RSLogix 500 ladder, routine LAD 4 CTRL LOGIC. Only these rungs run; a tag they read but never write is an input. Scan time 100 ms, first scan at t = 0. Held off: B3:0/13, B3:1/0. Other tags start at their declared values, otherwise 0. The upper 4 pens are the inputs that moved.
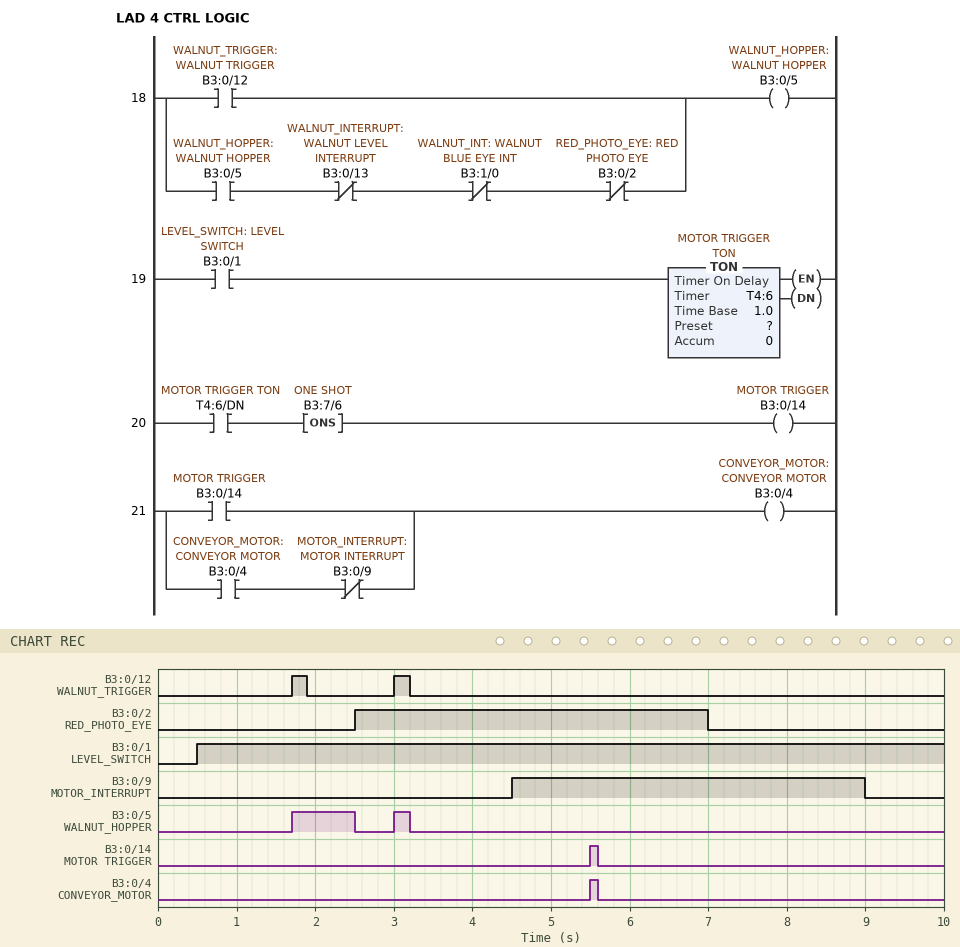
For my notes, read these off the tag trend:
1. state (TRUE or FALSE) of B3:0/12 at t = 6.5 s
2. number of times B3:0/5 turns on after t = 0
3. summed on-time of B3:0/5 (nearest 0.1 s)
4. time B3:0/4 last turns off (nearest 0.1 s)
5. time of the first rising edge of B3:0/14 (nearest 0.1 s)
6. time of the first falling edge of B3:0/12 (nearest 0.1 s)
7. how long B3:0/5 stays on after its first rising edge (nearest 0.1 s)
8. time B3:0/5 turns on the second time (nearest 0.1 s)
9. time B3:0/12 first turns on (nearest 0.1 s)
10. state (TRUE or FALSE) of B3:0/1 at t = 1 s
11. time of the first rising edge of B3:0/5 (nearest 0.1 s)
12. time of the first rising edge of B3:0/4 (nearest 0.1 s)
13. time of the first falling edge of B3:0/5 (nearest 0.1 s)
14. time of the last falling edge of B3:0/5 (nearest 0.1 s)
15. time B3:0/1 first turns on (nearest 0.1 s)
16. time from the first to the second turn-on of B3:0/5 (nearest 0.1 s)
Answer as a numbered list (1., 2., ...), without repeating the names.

1. FALSE
2. 2
3. 1.0 s
4. 5.6 s
5. 5.5 s
6. 1.9 s
7. 0.8 s
8. 3.0 s
9. 1.7 s
10. TRUE
11. 1.7 s
12. 5.5 s
13. 2.5 s
14. 3.2 s
15. 0.5 s
16. 1.3 s
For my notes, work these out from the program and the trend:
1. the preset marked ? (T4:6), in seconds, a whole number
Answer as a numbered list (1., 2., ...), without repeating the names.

1. 5 s
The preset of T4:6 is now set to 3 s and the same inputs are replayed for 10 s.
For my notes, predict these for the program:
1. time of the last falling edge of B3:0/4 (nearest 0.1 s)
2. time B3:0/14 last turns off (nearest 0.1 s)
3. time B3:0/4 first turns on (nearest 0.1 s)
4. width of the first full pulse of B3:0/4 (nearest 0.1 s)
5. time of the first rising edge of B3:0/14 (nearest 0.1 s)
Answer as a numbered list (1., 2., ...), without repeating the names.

1. 4.5 s
2. 3.6 s
3. 3.5 s
4. 1.0 s
5. 3.5 s
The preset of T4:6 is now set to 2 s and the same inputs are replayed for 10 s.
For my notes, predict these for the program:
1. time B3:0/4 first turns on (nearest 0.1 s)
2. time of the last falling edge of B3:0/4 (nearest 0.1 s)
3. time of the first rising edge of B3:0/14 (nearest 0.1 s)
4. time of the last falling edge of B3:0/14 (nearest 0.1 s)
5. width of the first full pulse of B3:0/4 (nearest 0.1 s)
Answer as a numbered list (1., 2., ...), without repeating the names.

1. 2.5 s
2. 4.5 s
3. 2.5 s
4. 2.6 s
5. 2.0 s
